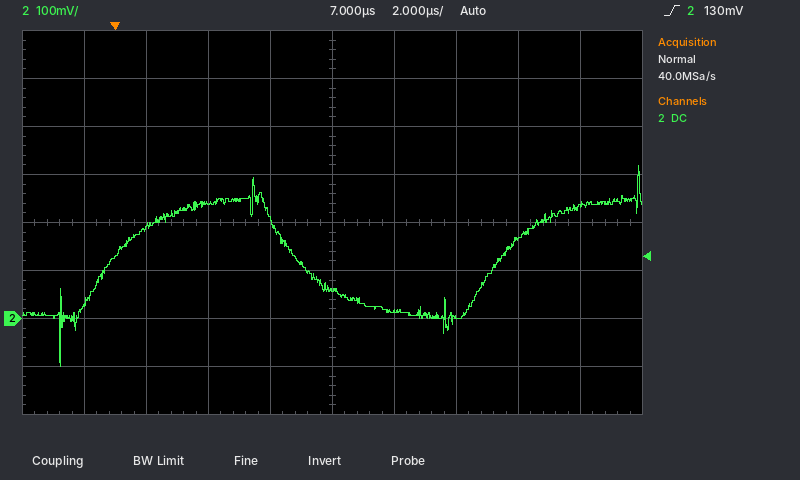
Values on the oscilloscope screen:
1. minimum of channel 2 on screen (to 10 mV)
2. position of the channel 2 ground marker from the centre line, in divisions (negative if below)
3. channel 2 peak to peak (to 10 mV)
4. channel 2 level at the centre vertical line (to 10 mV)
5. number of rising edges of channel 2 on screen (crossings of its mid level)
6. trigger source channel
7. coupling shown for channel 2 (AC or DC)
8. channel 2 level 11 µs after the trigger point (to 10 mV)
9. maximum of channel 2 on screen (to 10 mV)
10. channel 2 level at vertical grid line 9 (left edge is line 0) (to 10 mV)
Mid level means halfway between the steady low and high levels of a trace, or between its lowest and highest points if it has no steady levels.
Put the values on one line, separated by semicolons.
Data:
-100 mV; -2.0 div; 420 mV; 60 mV; 2; channel 2; DC; 0 mV; 320 mV; 230 mV
